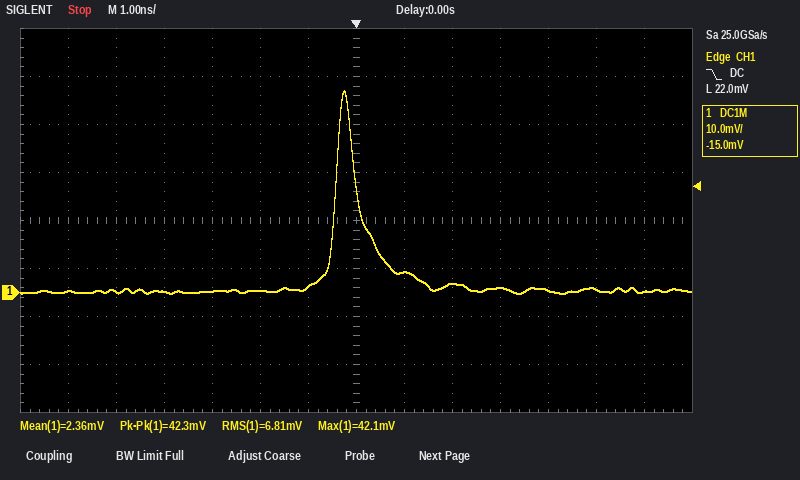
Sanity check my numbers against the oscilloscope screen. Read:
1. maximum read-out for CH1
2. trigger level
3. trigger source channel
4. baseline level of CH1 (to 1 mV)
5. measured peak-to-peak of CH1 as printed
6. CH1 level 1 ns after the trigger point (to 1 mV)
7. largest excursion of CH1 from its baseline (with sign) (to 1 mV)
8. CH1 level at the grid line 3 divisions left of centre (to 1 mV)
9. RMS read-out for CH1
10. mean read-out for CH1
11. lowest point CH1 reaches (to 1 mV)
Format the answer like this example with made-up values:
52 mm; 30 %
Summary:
42.1 mV; 22.0 mV; CH1; 0 mV; 42.3 mV; 4 mV; +42 mV; 0 mV; 6.81 mV; 2.36 mV; 0 mV
